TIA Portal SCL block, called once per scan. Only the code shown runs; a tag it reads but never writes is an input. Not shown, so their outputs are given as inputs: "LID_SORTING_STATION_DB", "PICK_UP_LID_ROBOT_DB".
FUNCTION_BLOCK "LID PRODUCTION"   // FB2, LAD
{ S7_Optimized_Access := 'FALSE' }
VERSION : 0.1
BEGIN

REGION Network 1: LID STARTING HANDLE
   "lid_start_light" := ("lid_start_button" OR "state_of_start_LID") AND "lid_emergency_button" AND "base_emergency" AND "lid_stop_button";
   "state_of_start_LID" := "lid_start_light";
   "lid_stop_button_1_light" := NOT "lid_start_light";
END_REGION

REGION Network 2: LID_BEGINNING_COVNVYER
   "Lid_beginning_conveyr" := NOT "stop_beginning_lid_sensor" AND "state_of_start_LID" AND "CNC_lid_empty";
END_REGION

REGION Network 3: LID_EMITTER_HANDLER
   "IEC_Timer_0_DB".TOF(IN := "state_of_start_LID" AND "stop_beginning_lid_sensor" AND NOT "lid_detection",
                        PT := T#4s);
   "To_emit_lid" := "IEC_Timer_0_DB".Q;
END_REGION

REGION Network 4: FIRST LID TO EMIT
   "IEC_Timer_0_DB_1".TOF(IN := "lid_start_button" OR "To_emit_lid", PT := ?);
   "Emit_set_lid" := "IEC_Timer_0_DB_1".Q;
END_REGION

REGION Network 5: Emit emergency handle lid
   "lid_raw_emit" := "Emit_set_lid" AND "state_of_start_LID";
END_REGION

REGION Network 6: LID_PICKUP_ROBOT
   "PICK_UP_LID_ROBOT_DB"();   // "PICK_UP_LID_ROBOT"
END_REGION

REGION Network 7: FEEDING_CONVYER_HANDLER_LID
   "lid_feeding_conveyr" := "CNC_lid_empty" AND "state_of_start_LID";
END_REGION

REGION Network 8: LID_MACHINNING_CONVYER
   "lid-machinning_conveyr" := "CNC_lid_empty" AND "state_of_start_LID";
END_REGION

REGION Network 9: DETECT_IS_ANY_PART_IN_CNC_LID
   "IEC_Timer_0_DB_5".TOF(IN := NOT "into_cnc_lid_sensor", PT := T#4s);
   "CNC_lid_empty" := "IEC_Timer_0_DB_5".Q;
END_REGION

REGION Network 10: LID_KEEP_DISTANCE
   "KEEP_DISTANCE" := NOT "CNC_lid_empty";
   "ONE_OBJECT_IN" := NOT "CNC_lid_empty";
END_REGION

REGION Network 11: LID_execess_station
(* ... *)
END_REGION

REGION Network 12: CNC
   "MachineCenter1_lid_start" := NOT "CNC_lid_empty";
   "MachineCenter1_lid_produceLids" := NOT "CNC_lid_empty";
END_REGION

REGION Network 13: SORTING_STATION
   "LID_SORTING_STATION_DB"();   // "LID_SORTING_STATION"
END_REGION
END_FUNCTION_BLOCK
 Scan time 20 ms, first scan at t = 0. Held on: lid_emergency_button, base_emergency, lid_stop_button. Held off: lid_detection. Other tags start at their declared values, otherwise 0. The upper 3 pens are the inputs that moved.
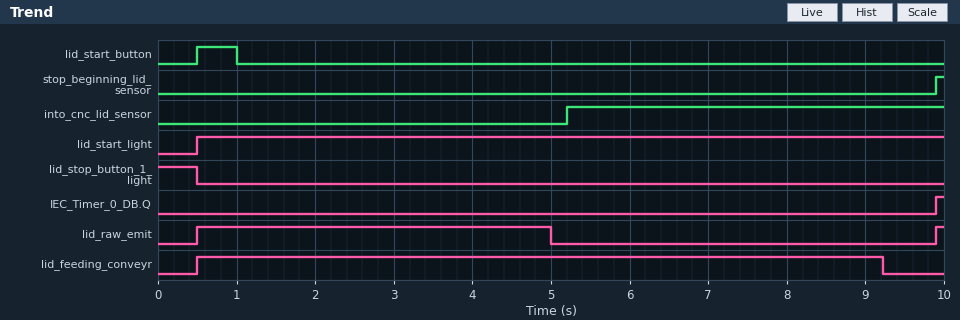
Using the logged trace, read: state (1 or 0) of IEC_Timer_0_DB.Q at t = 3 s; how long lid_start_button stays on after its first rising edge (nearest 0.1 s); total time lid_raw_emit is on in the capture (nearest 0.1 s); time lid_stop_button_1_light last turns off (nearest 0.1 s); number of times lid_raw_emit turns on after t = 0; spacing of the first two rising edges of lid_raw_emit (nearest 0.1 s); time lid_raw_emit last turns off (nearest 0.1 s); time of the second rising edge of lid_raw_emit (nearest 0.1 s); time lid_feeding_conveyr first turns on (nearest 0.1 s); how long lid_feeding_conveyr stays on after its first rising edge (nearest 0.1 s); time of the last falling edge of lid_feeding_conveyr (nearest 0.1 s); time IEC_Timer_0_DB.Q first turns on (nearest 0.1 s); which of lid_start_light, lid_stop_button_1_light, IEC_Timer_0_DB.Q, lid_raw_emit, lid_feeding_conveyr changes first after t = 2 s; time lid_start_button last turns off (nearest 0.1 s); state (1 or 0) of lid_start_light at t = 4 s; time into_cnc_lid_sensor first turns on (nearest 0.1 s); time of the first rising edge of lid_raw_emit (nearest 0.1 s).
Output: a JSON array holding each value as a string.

["0", "0.5 s", "4.6 s", "0.5 s", "2", "9.4 s", "5.0 s", "9.9 s", "0.5 s", "8.7 s", "9.2 s", "9.9 s", "lid_raw_emit", "1.0 s", "1", "5.2 s", "0.5 s"]
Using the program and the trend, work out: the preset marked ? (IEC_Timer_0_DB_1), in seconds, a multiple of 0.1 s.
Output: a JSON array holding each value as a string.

["4.0 s"]
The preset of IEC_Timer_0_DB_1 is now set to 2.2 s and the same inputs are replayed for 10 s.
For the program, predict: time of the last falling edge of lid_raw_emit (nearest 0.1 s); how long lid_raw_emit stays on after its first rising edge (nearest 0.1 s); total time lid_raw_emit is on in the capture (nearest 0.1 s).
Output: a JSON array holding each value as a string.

["3.2 s", "2.7 s", "2.8 s"]
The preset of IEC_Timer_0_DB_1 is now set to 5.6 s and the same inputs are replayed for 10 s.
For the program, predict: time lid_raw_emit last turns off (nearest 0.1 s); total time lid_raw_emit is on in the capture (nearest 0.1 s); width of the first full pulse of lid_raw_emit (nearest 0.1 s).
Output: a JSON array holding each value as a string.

["6.6 s", "6.2 s", "6.1 s"]
